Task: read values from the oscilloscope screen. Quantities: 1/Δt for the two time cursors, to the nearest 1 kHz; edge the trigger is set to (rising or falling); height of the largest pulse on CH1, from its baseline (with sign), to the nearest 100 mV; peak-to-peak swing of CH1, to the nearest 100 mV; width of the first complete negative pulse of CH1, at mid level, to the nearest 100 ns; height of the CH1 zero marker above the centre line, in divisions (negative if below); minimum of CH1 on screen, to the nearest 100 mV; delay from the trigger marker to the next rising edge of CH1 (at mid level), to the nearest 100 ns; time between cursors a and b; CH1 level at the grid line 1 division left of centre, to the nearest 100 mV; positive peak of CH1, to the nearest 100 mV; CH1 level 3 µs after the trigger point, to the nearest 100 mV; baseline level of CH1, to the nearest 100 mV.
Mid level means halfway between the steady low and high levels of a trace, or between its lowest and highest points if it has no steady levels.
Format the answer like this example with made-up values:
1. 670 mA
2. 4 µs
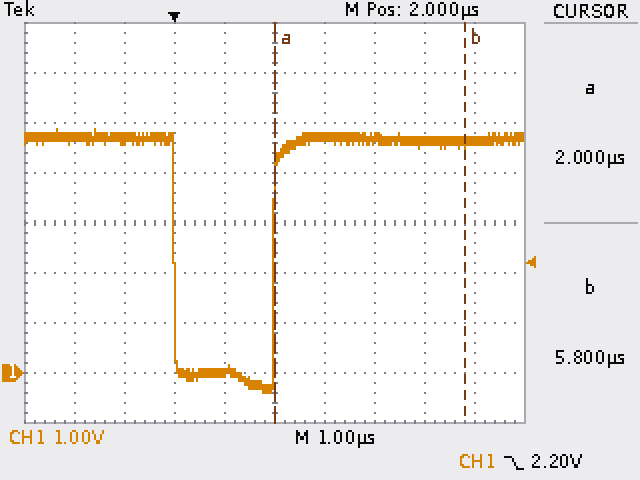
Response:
1. 263 kHz
2. falling
3. -5.1 V
4. 5.3 V
5. 2.0 µs
6. -3.0 div
7. -400 mV
8. 2.0 µs
9. 3.8 µs
10. 0.0 V
11. 4.9 V
12. 4.7 V
13. 4.7 V
